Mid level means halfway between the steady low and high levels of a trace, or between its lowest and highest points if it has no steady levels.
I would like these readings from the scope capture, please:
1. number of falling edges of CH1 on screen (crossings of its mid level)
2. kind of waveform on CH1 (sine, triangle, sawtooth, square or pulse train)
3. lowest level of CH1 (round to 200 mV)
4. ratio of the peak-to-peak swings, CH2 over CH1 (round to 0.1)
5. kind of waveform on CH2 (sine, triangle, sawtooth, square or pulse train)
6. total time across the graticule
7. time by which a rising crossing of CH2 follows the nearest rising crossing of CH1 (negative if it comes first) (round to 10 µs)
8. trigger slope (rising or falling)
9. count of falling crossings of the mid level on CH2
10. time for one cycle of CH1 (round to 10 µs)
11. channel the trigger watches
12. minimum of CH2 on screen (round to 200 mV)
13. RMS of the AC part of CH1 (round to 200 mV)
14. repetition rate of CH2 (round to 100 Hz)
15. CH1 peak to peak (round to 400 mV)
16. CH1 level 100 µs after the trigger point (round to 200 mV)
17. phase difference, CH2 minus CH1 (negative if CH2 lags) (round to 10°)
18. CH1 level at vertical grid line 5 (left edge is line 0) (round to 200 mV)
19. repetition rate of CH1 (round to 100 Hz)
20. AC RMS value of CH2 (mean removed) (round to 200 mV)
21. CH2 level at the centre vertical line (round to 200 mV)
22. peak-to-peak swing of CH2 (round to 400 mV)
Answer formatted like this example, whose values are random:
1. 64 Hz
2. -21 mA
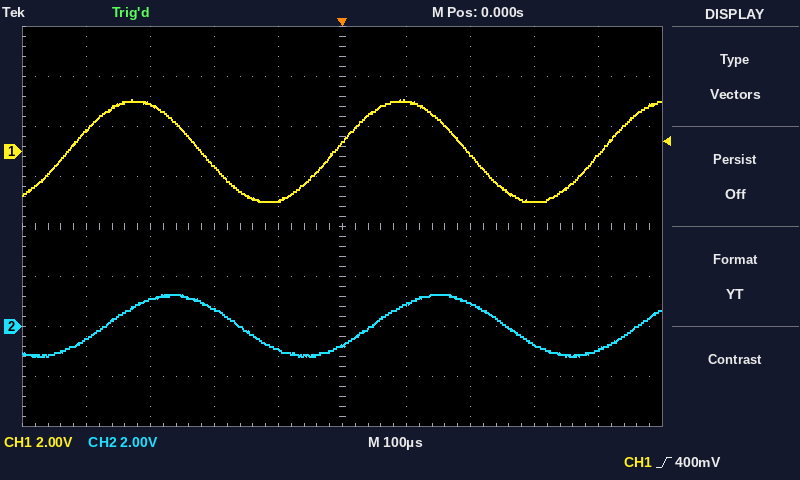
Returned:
1. 2
2. sine
3. -2.0 V
4. 0.6
5. sine
6. 1 ms
7. +60 µs
8. rising
9. 2
10. 420 µs
11. CH1
12. -1.2 V
13. 1.4 V
14. 2.4 kHz
15. 4.0 V
16. 2.0 V
17. -50°
18. 400 mV
19. 2.4 kHz
20. 800 mV
21. -800 mV
22. 2.4 V
